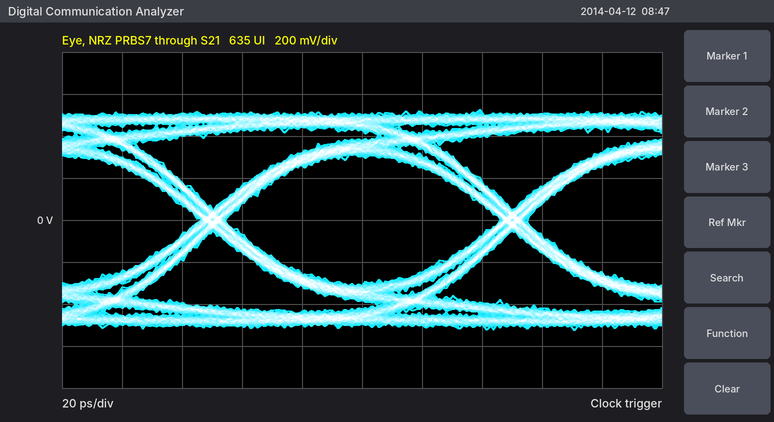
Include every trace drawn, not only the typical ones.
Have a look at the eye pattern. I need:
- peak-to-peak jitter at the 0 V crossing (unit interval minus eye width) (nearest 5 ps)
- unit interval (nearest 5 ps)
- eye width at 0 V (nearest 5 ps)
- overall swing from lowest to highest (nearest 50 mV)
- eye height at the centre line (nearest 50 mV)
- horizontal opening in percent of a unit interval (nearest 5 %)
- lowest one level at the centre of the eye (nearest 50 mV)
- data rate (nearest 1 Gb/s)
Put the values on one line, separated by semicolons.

10 ps; 100 ps; 90 ps; 1.05 V; 600 mV; 90 %; 300 mV; 10 Gb/s
